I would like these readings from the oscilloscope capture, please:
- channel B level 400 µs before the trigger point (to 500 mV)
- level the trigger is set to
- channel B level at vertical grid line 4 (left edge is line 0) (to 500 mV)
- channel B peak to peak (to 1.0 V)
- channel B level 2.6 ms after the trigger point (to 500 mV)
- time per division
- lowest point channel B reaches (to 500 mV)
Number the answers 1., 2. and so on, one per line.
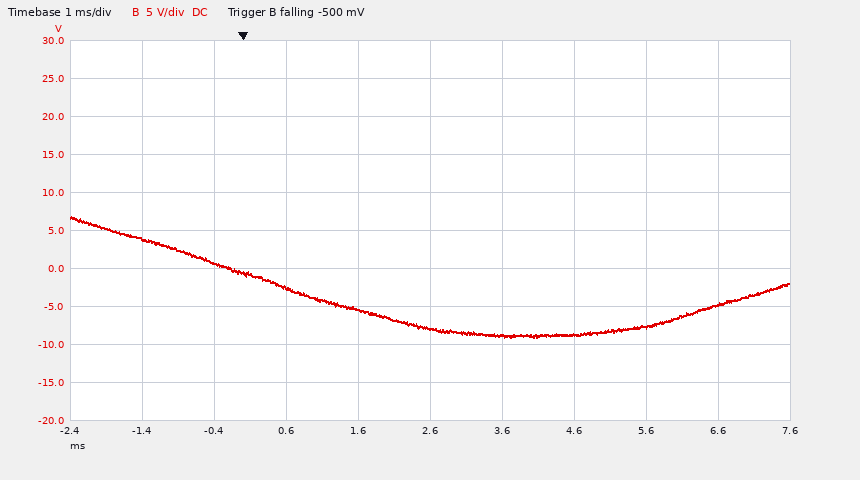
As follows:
1. 500 mV
2. -500 mV
3. -5.5 V
4. 16.0 V
5. -8.0 V
6. 1 ms
7. -9.0 V
